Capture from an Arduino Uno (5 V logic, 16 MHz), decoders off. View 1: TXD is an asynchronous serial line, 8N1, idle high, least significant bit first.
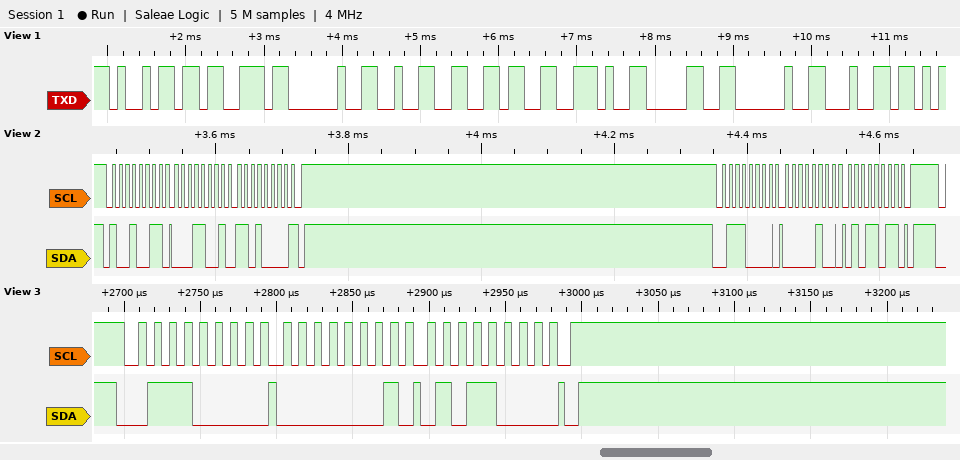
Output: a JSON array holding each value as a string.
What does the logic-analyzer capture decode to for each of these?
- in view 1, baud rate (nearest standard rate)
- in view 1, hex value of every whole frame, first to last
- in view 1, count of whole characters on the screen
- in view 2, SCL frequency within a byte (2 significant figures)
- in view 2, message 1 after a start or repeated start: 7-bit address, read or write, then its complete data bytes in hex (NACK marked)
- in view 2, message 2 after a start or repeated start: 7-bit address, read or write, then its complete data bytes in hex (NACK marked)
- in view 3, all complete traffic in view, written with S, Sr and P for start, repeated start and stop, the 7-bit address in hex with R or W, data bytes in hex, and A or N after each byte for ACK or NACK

["9600 baud", "69 73 20 32 36 2E 30 20 64", "9", "100 kHz", "0x49 read: 19 D0 NACK", "0x38 write: 04 5B", "S 38W A 01 A 58 A P"]
